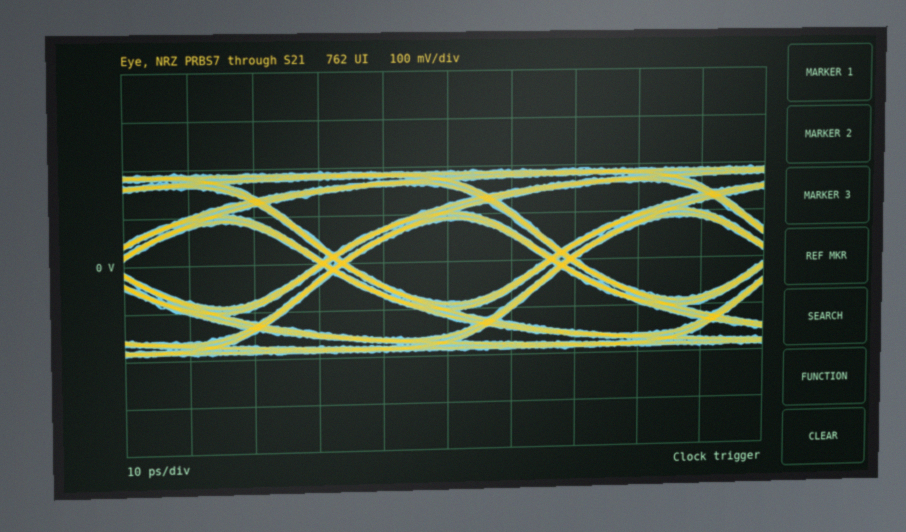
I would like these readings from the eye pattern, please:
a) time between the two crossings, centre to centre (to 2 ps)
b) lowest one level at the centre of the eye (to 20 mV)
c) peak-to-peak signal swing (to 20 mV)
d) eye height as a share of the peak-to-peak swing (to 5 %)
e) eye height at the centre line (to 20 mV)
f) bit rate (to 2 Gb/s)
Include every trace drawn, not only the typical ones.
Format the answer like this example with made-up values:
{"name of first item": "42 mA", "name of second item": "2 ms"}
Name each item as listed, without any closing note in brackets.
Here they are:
{"time between the two crossings, centre to centre": "36 ps", "lowest one level at the centre of the eye": "80 mV", "peak-to-peak signal swing": "380 mV", "eye height as a share of the peak-to-peak swing": "45 %", "eye height at the centre line": "180 mV", "bit rate": "28 Gb/s"}
